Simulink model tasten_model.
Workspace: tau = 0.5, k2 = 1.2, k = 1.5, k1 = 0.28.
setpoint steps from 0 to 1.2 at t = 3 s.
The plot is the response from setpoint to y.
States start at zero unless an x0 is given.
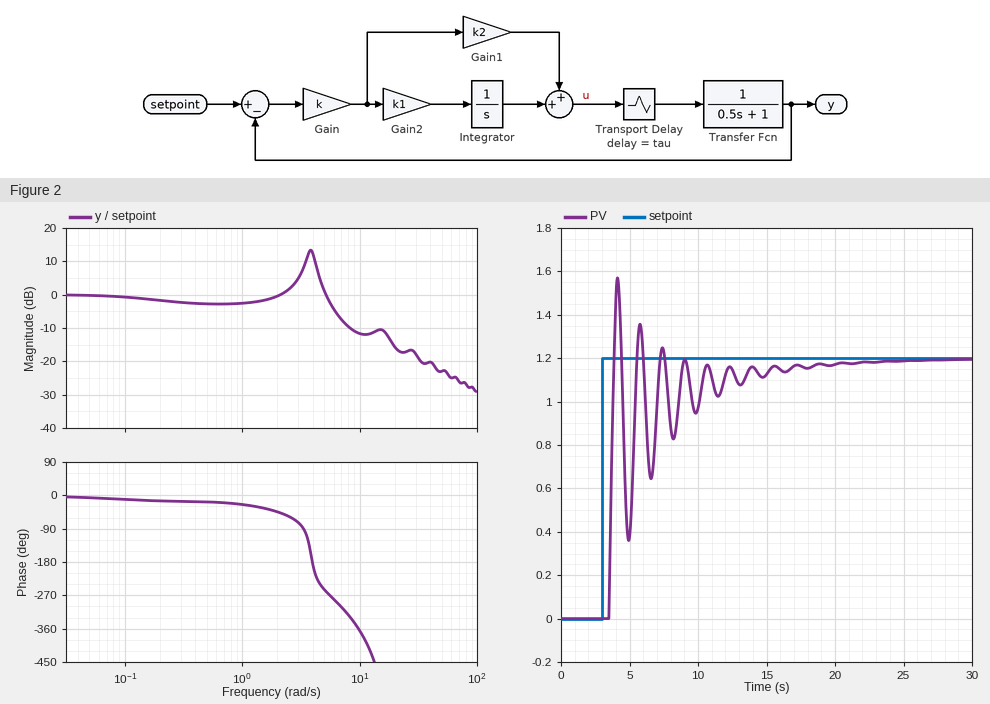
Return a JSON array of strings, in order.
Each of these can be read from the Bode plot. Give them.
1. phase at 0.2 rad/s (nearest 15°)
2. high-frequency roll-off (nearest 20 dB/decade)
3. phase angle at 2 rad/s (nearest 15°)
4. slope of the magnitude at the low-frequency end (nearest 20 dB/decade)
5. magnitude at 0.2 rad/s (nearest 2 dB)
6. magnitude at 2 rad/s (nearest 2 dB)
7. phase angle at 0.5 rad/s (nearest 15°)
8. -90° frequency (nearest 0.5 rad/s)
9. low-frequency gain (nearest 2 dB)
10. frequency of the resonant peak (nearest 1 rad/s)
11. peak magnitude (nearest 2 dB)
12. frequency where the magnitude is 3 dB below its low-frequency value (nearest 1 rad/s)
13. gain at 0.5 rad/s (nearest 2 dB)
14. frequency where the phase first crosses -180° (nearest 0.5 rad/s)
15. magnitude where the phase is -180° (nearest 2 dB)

["-15°", "-20 dB/decade", "-45°", "0 dB/decade", "-2 dB", "0 dB", "-15°", "3.5 rad/s", "0 dB", "4 rad/s", "14 dB", "6 rad/s", "-2 dB", "4.0 rad/s", "12 dB"]
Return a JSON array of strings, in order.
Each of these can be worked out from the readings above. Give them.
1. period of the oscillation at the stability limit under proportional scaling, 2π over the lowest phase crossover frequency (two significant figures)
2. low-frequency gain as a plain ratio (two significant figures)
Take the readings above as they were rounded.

["1.6 s", "1.0"]
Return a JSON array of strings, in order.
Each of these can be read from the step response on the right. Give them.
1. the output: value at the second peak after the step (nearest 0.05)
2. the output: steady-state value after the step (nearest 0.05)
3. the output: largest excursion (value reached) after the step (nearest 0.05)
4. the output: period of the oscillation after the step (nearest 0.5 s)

["1.35", "1.20", "1.55", "1.5 s"]
